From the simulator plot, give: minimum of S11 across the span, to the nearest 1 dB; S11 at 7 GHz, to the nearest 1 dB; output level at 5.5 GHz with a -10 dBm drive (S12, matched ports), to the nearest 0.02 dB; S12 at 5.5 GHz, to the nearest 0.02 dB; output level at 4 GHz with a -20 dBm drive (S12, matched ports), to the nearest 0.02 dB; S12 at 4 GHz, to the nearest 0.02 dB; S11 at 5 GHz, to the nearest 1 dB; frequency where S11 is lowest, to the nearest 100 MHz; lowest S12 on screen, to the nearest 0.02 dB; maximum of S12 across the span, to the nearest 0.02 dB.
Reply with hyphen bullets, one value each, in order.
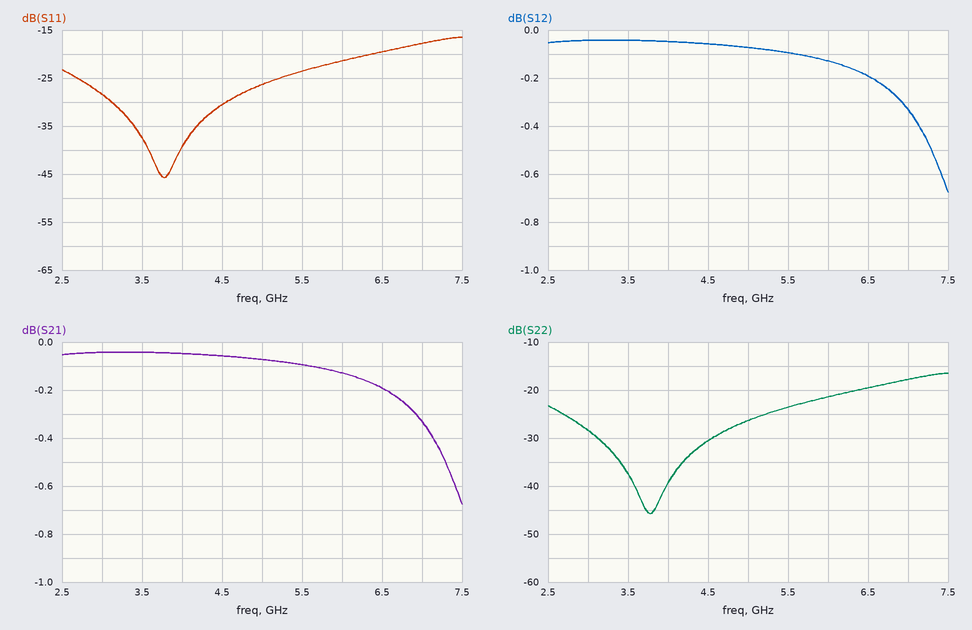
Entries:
- -46 dB
- -18 dB
- -10.10 dBm
- -0.10 dB
- -20.04 dBm
- -0.04 dB
- -26 dB
- 3.8 GHz
- -0.68 dB
- -0.04 dB
